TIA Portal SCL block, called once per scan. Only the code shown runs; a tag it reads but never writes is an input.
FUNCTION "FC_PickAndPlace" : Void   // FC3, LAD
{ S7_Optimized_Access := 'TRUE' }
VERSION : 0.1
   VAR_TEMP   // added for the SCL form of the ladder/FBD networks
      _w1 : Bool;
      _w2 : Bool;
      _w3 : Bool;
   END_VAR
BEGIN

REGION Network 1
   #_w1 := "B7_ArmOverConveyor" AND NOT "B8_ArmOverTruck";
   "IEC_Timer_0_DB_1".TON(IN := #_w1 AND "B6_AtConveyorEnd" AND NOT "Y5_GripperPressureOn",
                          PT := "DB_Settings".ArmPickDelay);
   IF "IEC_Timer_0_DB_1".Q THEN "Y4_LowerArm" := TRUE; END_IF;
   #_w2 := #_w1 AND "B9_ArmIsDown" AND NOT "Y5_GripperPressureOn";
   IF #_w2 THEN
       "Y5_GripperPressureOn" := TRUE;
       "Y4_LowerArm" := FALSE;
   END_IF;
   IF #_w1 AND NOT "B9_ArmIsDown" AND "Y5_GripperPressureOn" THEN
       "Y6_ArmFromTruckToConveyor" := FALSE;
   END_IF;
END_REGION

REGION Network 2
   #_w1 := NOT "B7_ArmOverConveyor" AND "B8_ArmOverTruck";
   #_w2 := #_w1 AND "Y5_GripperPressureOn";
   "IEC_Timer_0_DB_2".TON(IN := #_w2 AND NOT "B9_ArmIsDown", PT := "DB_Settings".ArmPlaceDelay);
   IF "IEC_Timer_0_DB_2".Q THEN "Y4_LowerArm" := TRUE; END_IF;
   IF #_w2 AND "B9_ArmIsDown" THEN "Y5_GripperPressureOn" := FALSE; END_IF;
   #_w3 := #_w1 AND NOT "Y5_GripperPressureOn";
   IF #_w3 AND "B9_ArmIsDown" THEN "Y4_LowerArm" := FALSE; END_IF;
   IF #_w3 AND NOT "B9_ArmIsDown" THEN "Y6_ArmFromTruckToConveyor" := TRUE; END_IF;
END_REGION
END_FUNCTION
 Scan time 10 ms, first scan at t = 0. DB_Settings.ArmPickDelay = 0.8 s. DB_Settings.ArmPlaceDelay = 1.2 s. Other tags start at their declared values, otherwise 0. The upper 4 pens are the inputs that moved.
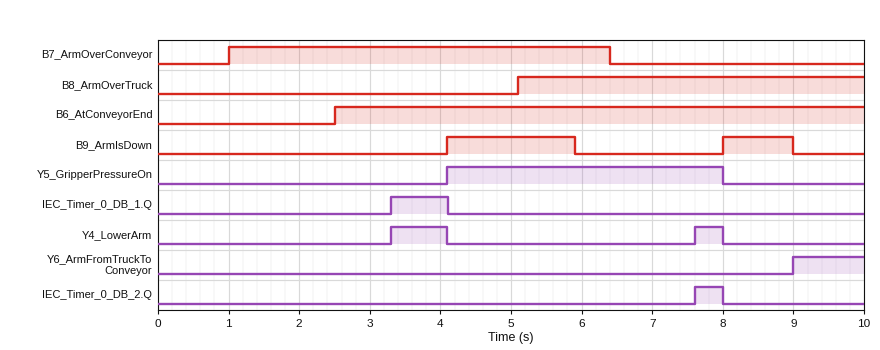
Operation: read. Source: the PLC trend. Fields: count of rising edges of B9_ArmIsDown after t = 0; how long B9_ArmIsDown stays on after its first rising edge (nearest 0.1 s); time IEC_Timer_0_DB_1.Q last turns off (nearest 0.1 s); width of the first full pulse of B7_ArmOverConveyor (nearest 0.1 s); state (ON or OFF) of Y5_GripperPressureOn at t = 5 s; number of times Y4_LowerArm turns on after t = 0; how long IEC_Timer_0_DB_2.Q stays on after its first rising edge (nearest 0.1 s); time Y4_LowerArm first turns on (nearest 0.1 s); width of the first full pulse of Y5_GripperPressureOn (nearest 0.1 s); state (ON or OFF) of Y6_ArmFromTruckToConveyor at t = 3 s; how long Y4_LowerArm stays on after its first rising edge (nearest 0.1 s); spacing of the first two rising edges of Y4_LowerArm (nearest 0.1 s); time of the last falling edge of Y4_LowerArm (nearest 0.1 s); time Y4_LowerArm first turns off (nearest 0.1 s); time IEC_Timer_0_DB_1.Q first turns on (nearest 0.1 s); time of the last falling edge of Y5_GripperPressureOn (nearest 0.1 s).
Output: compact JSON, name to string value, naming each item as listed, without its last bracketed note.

{"count of rising edges of B9_ArmIsDown after t = 0": "2", "how long B9_ArmIsDown stays on after its first rising edge": "1.8 s", "time IEC_Timer_0_DB_1.Q last turns off": "4.1 s", "width of the first full pulse of B7_ArmOverConveyor": "5.4 s", "state (ON or OFF) of Y5_GripperPressureOn at t = 5 s": "ON", "number of times Y4_LowerArm turns on after t = 0": "2", "how long IEC_Timer_0_DB_2.Q stays on after its first rising edge": "0.4 s", "time Y4_LowerArm first turns on": "3.3 s", "width of the first full pulse of Y5_GripperPressureOn": "3.9 s", "state (ON or OFF) of Y6_ArmFromTruckToConveyor at t = 3 s": "OFF", "how long Y4_LowerArm stays on after its first rising edge": "0.8 s", "spacing of the first two rising edges of Y4_LowerArm": "4.3 s", "time of the last falling edge of Y4_LowerArm": "8.0 s", "time Y4_LowerArm first turns off": "4.1 s", "time IEC_Timer_0_DB_1.Q first turns on": "3.3 s", "time of the last falling edge of Y5_GripperPressureOn": "8.0 s"}
